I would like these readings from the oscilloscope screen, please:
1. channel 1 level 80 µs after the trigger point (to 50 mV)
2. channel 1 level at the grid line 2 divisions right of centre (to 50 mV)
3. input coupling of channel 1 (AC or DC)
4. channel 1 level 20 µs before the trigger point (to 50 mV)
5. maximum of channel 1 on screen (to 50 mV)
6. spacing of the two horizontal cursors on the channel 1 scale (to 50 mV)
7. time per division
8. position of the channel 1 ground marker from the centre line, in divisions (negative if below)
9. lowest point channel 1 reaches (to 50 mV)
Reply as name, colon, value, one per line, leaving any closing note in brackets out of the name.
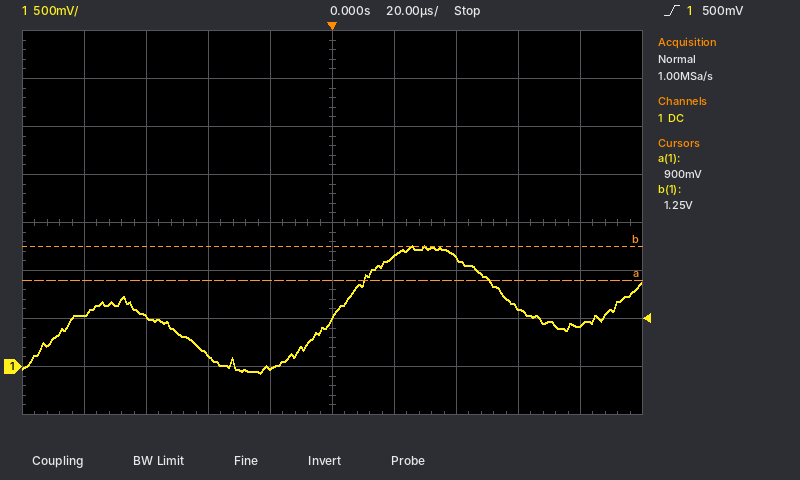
channel 1 level 80 µs after the trigger point: 450 mV
channel 1 level at the grid line 2 divisions right of centre: 1.15 V
input coupling of channel 1: DC
channel 1 level 20 µs before the trigger point: 0 mV
maximum of channel 1 on screen: 1.25 V
spacing of the two horizontal cursors on the channel 1 scale: 350 mV
time per division: 20 µs
position of the channel 1 ground marker from the centre line, in divisions: -3.0 div
lowest point channel 1 reaches: -50 mV
